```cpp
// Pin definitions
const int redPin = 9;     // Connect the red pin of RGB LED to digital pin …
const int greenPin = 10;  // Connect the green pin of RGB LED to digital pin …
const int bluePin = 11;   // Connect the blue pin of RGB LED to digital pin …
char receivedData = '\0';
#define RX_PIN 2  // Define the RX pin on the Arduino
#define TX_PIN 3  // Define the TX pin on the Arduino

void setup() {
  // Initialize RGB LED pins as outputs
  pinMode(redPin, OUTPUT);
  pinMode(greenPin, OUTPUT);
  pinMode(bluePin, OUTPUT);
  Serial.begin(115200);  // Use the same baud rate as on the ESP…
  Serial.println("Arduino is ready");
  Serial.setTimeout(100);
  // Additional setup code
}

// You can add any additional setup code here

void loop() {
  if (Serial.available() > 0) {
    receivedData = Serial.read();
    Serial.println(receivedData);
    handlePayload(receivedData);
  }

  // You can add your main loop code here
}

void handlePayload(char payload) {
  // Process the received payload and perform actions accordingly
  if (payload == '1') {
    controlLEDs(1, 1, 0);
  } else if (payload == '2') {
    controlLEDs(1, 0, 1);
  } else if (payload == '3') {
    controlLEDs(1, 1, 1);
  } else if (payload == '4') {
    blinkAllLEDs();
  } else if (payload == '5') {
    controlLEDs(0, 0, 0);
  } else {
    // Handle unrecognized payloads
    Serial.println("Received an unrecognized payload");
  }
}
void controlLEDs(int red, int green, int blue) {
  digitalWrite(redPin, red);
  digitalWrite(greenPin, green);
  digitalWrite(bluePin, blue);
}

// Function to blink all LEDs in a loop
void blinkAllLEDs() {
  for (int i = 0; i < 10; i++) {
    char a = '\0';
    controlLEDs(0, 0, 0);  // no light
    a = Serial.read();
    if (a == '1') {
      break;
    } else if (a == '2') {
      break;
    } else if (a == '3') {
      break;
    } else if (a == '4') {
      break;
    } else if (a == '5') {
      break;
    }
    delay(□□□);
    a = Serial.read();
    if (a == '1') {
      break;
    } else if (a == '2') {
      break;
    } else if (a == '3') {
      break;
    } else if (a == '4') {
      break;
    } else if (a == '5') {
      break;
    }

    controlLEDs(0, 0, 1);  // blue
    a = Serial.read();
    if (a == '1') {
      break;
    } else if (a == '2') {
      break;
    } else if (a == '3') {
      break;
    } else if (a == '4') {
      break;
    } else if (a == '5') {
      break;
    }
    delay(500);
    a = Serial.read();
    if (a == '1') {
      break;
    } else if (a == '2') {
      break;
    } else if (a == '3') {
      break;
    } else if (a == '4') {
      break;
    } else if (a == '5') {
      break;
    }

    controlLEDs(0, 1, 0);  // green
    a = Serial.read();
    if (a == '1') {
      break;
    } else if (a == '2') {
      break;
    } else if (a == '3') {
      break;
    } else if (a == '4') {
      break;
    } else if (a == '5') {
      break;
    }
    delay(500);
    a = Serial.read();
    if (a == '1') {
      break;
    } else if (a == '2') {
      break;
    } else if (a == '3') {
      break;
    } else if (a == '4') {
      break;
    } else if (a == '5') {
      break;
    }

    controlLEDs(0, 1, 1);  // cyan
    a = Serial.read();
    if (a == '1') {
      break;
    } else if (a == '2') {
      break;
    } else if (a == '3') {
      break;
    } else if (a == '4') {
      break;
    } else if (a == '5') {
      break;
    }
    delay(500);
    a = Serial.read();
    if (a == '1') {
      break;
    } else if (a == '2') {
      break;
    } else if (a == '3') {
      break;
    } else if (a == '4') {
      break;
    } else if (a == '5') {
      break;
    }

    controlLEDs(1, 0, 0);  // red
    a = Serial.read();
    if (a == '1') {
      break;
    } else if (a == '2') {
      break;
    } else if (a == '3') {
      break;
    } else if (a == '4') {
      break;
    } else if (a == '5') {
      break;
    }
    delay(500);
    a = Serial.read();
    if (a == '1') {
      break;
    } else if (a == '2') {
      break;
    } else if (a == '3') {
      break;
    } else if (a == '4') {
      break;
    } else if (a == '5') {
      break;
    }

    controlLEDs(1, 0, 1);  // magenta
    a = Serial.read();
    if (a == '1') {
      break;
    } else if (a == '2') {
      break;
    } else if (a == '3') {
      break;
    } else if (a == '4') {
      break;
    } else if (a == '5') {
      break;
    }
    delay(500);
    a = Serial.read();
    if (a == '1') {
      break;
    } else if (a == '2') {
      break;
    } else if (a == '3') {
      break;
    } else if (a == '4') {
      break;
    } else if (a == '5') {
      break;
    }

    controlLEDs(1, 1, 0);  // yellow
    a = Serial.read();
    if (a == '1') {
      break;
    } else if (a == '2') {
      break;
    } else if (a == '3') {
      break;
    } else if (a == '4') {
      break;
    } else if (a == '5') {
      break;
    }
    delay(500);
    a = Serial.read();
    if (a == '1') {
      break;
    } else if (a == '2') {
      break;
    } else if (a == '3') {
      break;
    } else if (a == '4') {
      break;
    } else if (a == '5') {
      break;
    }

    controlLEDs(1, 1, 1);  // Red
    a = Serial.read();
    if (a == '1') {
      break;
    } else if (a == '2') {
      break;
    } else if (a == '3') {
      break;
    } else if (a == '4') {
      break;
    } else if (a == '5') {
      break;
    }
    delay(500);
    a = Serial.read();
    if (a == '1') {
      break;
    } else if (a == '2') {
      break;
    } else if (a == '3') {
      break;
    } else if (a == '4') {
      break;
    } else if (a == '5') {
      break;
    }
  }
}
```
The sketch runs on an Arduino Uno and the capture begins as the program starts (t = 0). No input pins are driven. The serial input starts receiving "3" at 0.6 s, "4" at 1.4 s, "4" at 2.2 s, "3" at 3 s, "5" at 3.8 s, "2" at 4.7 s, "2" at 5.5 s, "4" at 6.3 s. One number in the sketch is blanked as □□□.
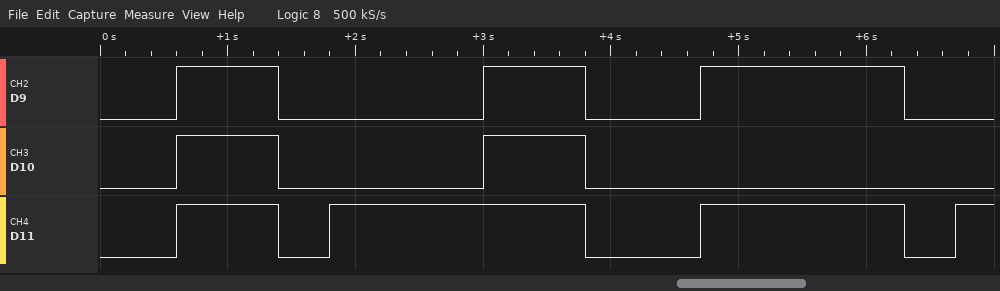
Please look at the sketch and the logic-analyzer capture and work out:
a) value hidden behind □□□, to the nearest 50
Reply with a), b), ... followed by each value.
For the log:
a) 400
